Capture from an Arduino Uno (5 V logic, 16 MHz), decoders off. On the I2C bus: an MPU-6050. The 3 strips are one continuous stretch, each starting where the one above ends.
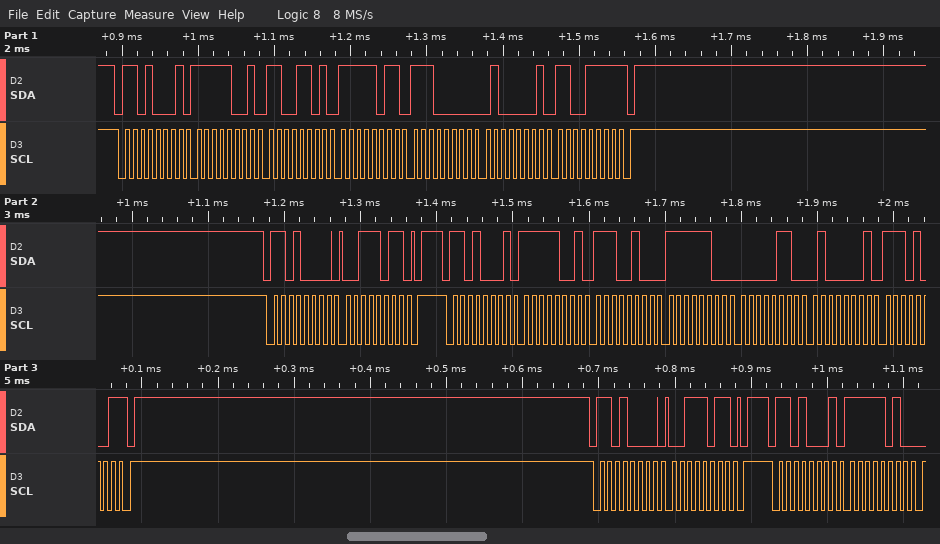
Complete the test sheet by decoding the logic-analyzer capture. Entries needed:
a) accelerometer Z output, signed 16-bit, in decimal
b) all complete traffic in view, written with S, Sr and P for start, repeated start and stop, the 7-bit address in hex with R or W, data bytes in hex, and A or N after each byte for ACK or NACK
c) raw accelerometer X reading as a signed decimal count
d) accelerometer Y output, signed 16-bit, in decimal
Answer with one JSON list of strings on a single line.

["16873", "S 68R A F9 A CD A FB A E0 A 41 A CF N P S 68W A 3B A P S 68R A F9 A E4 A FC A 06 A 41 A E9 N P S 68W A 3B A P S 68R A FA A", "-1564", "-1018"]
